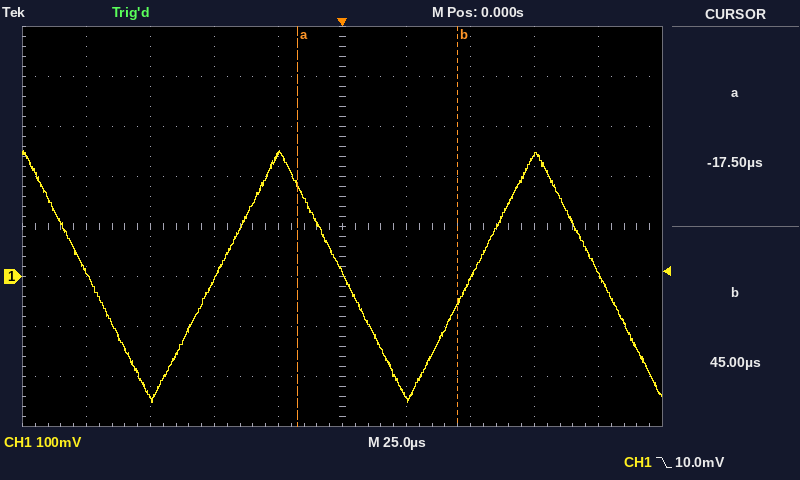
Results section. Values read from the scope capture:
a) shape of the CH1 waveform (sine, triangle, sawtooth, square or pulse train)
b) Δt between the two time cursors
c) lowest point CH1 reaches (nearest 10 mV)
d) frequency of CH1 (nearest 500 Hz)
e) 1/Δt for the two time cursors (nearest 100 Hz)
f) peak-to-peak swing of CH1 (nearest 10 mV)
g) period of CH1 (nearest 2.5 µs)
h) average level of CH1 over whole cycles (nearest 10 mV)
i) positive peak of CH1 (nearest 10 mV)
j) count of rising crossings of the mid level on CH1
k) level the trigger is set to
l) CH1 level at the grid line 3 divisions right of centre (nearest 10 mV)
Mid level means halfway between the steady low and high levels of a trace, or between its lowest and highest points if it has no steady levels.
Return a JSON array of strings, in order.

["triangle", "62.5 µs", "-250 mV", "10.0 kHz", "16.0 kHz", "500 mV", "100.0 µs", "0 mV", "250 mV", "2", "10.0 mV", "240 mV"]
